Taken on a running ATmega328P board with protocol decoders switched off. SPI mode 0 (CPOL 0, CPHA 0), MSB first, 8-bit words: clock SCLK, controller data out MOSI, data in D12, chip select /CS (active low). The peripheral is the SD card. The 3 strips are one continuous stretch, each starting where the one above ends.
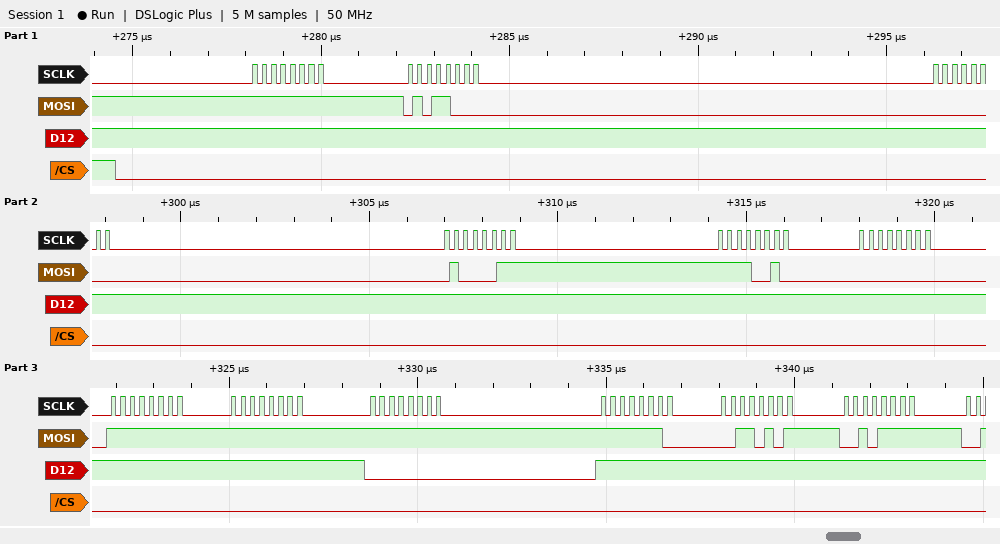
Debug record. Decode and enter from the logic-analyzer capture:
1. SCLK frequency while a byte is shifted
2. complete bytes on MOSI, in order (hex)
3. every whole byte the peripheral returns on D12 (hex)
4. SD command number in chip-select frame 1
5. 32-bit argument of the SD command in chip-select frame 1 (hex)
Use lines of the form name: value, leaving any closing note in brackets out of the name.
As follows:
SCLK frequency while a byte is shifted: 4 MHz
complete bytes on MOSI, in order: 0xFF 0x58 0x00 0x43 0xF2 0x00 0xFF 0xFF 0xFF 0xFE 0x35 0x2F
every whole byte the peripheral returns on D12: 0xFF 0xFF 0xFF 0xFF 0xFF 0xFF 0xFF 0xFF 0x00 0xFF 0xFF 0xFF
SD command number in chip-select frame 1: CMD24
32-bit argument of the SD command in chip-select frame 1: 0x0043F200
